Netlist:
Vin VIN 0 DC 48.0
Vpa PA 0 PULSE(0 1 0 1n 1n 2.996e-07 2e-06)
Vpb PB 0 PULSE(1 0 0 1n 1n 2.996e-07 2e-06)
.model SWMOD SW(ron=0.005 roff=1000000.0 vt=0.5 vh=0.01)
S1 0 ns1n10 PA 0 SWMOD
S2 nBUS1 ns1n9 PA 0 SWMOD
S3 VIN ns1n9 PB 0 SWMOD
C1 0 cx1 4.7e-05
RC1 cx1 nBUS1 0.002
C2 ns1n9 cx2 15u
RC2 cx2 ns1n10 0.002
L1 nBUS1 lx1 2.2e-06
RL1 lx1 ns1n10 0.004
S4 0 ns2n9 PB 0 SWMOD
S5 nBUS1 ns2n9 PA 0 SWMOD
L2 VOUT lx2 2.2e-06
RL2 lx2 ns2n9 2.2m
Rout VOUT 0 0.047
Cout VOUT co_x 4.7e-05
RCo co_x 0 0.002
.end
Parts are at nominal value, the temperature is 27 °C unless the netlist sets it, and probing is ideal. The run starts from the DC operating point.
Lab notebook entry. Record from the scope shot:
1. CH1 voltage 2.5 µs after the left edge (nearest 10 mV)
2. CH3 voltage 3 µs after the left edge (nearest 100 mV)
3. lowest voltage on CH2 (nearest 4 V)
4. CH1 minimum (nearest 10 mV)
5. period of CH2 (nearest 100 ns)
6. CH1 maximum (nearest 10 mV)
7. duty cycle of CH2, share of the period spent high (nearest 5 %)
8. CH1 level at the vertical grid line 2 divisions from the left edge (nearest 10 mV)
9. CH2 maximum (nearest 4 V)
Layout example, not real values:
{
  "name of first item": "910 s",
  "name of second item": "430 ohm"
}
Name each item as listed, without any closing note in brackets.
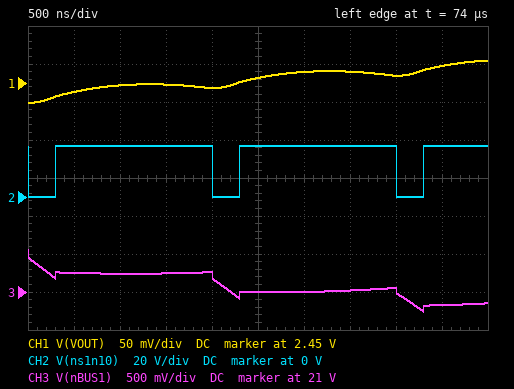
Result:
{
  "CH1 voltage 2.5 µs after the left edge": "2.46 V",
  "CH3 voltage 3 µs after the left edge": "21.0 V",
  "lowest voltage on CH2": "0 V",
  "CH1 minimum": "2.42 V",
  "period of CH2": "2.0 µs",
  "CH1 maximum": "2.48 V",
  "duty cycle of CH2, share of the period spent high": "85 %",
  "CH1 level at the vertical grid line 2 divisions from the left edge": "2.45 V",
  "CH2 maximum": "28 V"
}
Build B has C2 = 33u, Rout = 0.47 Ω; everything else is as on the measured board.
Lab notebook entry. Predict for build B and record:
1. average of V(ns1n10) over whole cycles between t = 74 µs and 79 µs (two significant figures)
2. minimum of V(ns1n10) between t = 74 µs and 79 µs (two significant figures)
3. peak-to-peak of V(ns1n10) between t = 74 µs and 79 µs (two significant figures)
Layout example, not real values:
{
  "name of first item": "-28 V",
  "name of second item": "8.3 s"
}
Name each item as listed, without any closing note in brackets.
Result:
{
  "average of V(ns1n10) over whole cycles between t = 74 µs and 79 µs": "22 V",
  "minimum of V(ns1n10) between t = 74 µs and 79 µs": "-74 mV",
  "peak-to-peak of V(ns1n10) between t = 74 µs and 79 µs": "26 V"
}
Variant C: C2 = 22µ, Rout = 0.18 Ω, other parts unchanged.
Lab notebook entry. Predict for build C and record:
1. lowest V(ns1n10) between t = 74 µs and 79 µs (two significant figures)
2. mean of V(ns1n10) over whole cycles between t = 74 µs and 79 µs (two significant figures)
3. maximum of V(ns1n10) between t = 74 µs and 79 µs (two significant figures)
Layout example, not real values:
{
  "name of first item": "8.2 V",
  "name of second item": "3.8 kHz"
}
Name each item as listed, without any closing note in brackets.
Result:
{
  "lowest V(ns1n10) between t = 74 µs and 79 µs": "-14 mV",
  "mean of V(ns1n10) over whole cycles between t = 74 µs and 79 µs": "22 V",
  "maximum of V(ns1n10) between t = 74 µs and 79 µs": "26 V"
}
